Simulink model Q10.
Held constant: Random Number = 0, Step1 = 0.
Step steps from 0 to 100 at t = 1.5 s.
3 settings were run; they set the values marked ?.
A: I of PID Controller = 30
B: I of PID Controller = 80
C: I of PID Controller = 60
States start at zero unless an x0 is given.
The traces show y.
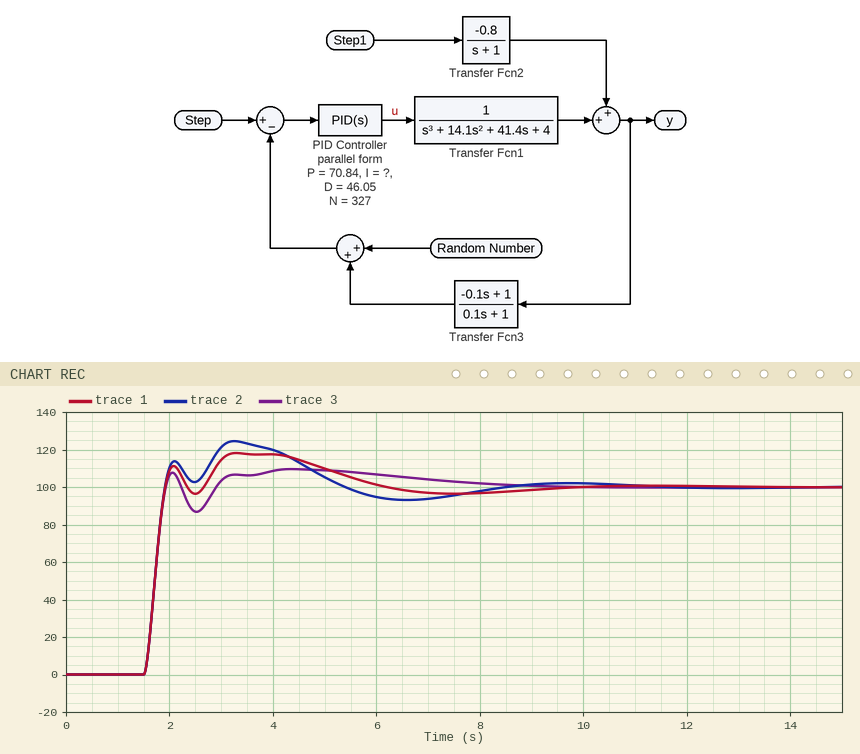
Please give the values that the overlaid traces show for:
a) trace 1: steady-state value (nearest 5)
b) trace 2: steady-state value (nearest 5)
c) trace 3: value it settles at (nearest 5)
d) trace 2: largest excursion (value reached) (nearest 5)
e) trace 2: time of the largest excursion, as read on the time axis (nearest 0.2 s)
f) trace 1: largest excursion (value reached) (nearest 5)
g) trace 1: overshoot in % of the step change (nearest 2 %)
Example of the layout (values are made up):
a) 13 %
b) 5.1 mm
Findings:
a) 100
b) 100
c) 100
d) 125
e) 3.2 s
f) 120
g) 18 %
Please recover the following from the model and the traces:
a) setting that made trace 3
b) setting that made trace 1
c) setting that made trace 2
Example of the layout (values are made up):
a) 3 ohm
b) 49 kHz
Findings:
a) A
b) C
c) B
